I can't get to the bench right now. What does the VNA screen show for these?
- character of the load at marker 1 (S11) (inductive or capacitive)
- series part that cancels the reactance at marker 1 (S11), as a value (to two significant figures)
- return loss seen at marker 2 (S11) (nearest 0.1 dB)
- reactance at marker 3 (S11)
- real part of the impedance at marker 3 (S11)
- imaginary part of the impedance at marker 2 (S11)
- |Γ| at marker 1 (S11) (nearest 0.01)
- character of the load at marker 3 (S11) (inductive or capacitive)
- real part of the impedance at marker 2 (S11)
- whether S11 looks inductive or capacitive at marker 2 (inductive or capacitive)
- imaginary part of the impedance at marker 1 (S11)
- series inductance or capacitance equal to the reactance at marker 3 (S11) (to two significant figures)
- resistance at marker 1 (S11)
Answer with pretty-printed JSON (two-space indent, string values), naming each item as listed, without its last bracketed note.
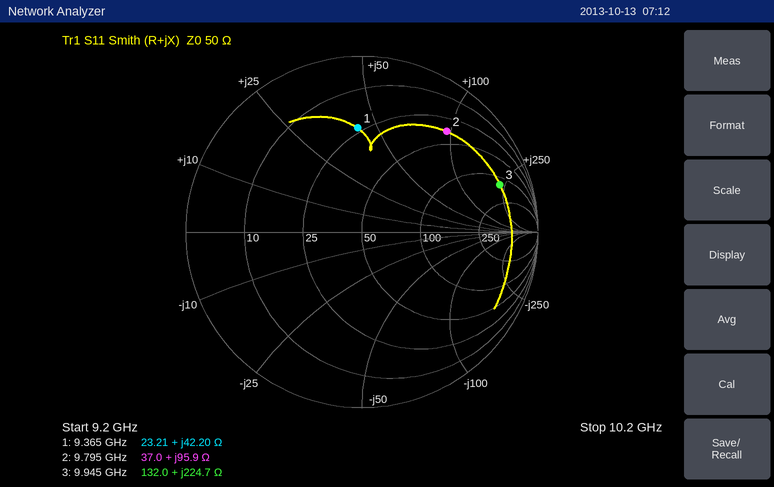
{
  "character of the load at marker 1 (S11)": "inductive",
  "series part that cancels the reactance at marker 1 (S11), as a value": "400 fF",
  "return loss seen at marker 2 (S11)": "2.5 dB",
  "reactance at marker 3": "+224.7 Ω",
  "real part of the impedance at marker 3": "132.0 Ω",
  "imaginary part of the impedance at marker 2": "+95.9 Ω",
  "|Γ| at marker 1 (S11)": "0.59",
  "character of the load at marker 3 (S11)": "inductive",
  "real part of the impedance at marker 2": "37.0 Ω",
  "whether S11 looks inductive or capacitive at marker 2": "inductive",
  "imaginary part of the impedance at marker 1": "+42.20 Ω",
  "series inductance or capacitance equal to the reactance at marker 3 (S11)": "3.6 nH",
  "resistance at marker 1": "23.21 Ω"
}
